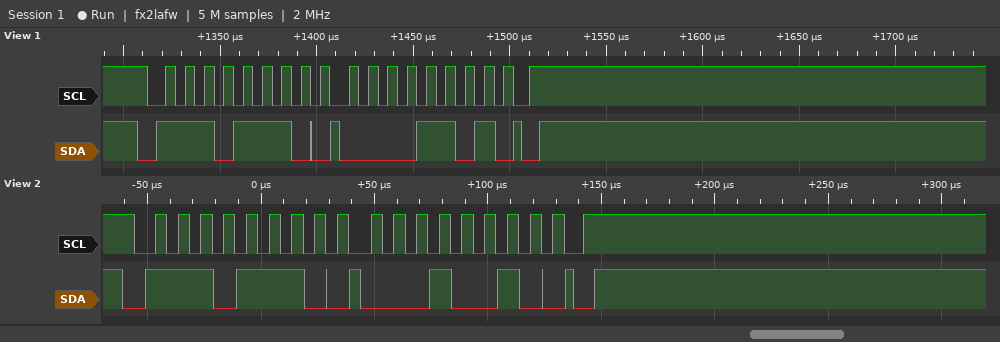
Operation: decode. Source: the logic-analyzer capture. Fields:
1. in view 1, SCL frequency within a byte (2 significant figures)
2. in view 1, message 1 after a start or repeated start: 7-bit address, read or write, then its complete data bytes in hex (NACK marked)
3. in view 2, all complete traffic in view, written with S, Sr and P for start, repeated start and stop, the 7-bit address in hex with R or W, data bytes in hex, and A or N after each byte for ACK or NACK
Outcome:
100 kHz
0x77 write: 0D
S 77W A 12 A P
